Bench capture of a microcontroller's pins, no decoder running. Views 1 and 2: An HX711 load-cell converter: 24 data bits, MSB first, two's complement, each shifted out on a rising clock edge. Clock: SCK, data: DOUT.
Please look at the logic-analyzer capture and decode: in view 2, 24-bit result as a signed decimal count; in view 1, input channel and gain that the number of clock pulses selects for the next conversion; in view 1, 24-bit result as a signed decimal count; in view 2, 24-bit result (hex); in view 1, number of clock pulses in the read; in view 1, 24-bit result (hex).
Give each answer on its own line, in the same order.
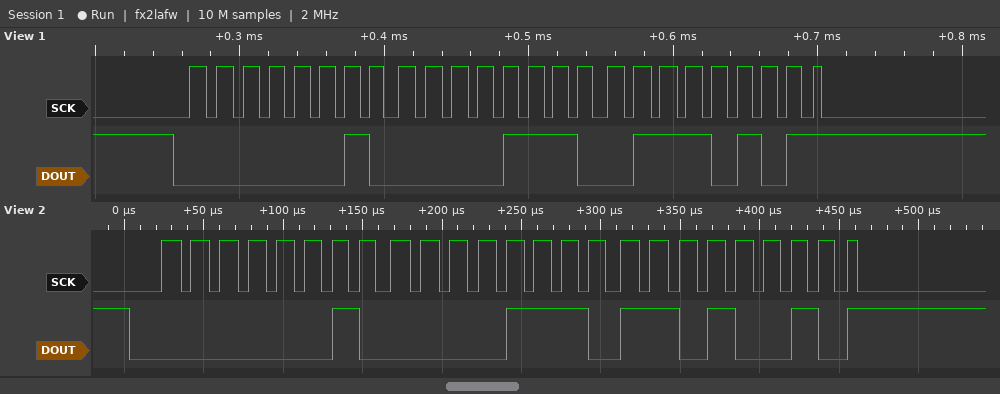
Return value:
134866
channel A, gain 128
134773
0x020ED2
25
0x020E75
